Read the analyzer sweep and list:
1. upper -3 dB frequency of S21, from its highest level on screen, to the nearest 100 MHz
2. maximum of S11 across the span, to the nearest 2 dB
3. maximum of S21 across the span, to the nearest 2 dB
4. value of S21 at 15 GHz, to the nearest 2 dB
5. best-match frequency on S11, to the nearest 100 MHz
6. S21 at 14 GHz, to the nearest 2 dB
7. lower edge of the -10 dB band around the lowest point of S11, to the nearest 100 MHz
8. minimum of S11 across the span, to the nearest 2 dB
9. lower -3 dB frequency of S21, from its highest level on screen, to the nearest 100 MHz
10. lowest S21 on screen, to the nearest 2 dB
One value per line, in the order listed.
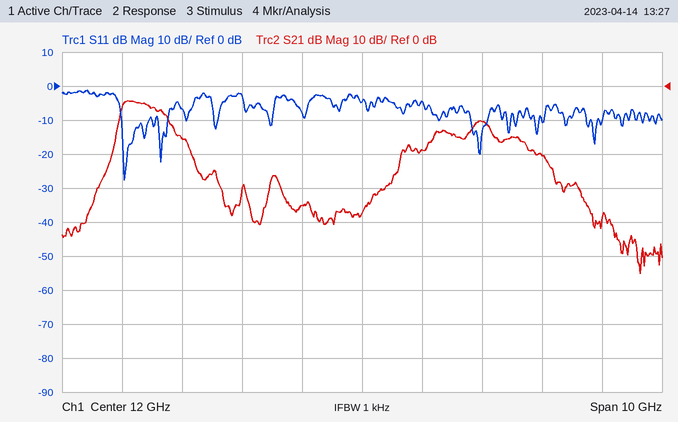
8.6 GHz
-2 dB
-4 dB
-20 dB
8.0 GHz
-10 dB
8.0 GHz
-28 dB
8.0 GHz
-56 dB
